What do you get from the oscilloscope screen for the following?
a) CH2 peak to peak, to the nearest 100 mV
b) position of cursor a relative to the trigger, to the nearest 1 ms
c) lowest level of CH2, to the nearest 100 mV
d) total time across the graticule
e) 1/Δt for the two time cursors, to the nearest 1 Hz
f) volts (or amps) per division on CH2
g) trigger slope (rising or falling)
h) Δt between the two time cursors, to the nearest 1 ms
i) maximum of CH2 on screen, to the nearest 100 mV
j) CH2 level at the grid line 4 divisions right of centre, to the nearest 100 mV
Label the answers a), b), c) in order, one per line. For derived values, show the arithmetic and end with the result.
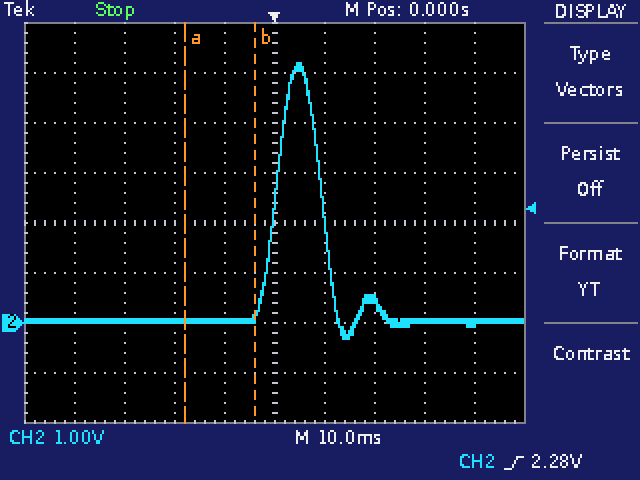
a) 5.2 V − (-300 mV) = 5.5 V
b) -18 ms
c) -300 mV
d) 100 ms
e) 1 / 14 ms ≈ 71 Hz
f) 1 V
g) rising
h) 14 ms
i) 5.2 V
j) 0.0 V
